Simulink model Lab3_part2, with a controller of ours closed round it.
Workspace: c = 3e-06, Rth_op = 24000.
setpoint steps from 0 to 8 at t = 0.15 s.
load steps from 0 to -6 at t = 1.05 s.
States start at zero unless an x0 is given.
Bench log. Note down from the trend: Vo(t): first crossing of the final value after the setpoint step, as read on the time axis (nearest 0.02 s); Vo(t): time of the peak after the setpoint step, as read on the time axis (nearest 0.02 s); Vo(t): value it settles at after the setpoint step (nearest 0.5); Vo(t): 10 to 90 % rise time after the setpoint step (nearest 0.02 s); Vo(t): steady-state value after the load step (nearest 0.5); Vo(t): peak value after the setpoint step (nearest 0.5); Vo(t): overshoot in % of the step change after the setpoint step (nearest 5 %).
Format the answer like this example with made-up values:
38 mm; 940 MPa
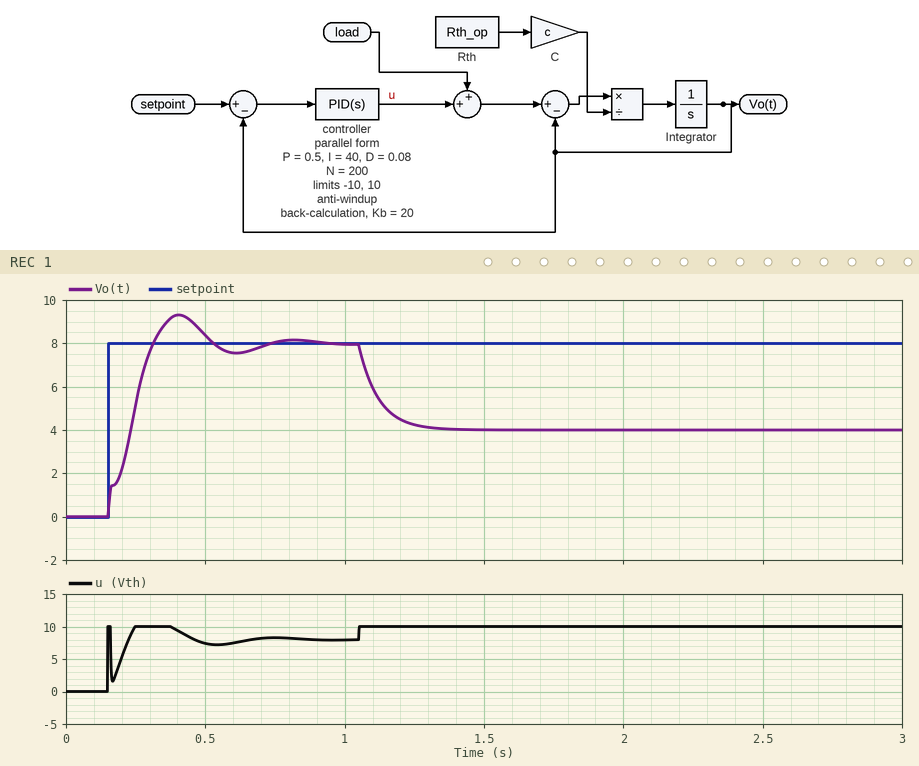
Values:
0.32 s; 0.40 s; 8.0; 0.14 s; 4.0; 9.5; 15 %
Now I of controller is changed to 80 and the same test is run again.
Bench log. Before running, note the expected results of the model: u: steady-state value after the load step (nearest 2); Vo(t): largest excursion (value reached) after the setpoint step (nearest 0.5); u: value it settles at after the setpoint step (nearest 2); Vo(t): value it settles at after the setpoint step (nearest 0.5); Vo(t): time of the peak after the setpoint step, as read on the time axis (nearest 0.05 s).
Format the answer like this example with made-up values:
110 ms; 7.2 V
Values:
10; 9.0; 8; 8.0; 0.35 s
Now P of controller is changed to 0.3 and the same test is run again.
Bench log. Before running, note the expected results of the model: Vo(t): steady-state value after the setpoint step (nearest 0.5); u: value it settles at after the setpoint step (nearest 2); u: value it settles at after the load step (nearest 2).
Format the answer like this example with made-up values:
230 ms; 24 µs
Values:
8.0; 8; 10
